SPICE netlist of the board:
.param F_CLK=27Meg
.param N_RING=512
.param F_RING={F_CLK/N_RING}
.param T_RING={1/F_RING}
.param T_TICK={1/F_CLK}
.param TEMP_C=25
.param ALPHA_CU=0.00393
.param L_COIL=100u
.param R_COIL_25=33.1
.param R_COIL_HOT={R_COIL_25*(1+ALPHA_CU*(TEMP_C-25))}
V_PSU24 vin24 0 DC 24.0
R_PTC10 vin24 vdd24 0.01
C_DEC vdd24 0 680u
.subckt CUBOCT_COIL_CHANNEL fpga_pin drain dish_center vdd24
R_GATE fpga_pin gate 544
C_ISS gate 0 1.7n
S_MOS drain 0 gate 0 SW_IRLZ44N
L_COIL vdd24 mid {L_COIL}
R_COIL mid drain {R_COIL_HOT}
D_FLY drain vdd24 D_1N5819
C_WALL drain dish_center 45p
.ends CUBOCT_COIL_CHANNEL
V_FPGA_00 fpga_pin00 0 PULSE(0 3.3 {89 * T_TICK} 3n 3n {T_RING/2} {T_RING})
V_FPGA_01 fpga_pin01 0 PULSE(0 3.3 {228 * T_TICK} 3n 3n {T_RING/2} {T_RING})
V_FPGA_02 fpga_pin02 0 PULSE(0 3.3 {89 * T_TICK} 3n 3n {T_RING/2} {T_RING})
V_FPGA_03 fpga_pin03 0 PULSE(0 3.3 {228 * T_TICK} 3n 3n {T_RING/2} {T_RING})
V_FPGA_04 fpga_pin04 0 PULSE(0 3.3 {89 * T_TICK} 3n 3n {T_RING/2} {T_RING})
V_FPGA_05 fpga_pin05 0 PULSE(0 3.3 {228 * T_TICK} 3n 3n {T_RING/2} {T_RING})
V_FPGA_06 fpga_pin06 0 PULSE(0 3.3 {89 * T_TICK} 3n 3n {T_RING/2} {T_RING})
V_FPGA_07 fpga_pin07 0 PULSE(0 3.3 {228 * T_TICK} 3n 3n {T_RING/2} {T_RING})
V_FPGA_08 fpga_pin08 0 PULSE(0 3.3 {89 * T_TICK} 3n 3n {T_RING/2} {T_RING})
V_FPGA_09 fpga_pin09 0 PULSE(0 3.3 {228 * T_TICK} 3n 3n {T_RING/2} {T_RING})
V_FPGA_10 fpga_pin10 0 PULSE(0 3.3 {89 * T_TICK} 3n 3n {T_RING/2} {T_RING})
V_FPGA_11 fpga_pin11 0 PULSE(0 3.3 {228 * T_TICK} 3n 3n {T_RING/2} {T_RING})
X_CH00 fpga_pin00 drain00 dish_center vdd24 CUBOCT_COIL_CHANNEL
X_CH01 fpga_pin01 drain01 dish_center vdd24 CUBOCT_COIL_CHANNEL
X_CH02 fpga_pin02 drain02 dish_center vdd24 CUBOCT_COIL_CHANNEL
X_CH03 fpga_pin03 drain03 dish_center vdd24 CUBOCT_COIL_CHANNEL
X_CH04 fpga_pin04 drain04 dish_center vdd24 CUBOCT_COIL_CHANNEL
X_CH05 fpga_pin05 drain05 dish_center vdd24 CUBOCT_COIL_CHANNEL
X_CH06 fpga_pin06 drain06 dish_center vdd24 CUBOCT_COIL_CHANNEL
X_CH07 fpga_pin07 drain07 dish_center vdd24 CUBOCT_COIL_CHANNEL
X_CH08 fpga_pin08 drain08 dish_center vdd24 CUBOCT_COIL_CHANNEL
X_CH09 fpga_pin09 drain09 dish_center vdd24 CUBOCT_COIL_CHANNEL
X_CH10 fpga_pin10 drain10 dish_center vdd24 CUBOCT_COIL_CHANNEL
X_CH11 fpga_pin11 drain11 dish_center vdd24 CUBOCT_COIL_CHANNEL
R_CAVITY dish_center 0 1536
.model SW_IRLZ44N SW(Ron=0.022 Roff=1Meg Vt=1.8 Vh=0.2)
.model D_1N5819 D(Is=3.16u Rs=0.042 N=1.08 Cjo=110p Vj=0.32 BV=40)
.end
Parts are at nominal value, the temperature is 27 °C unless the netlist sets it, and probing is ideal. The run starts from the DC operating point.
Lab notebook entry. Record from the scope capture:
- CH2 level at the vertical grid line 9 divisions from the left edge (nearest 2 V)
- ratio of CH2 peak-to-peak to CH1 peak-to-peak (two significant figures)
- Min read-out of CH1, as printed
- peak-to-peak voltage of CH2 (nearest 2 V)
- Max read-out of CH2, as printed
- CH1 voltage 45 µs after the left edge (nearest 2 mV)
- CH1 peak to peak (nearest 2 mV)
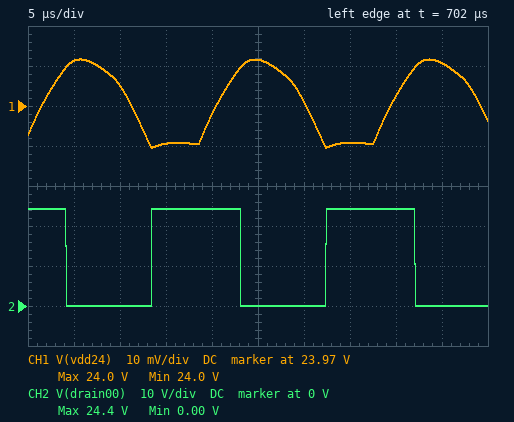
0 V
1100
24.0 V
24 V
24.4 V
23.980 V
22 mV
